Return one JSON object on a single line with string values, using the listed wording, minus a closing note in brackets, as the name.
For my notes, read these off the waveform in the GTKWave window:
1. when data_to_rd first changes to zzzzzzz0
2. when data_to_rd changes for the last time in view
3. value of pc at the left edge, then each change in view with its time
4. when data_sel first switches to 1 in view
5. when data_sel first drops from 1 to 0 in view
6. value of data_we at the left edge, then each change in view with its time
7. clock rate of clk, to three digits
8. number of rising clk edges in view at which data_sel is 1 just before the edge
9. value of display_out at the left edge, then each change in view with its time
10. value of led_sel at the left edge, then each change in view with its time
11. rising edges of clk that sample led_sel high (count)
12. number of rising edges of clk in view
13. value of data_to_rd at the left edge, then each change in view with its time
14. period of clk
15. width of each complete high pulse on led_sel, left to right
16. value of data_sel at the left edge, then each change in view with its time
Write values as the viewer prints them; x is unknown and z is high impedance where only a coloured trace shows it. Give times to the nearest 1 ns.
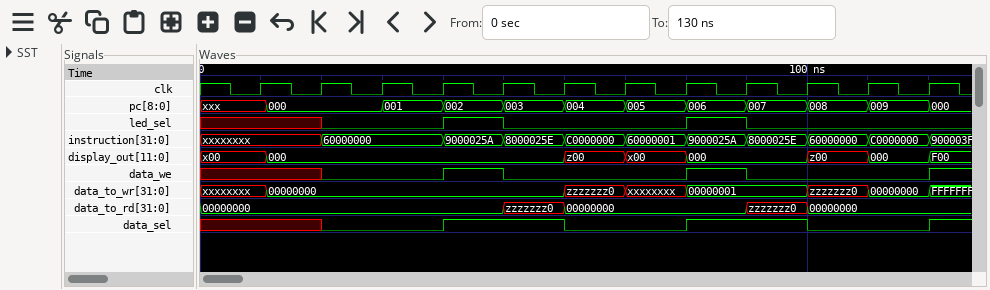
{"when data_to_rd first changes to zzzzzzz0": "50 ns", "when data_to_rd changes for the last time in view": "100 ns", "value of pc at the left edge, then each change in view with its time": "xxx, 000 at 11 ns, 001 at 30 ns, 002 at 40 ns, 003 at 50 ns, 004 at 60 ns, 005 at 70 ns, 006 at 80 ns, 007 at 90 ns, 008 at 100 ns, 009 at 110 ns, 000 at 120 ns", "when data_sel first switches to 1 in view": "40 ns", "when data_sel first drops from 1 to 0 in view": "60 ns", "value of data_we at the left edge, then each change in view with its time": "x, 0 at 20 ns, 1 at 40 ns, 0 at 50 ns, 1 at 80 ns, 0 at 90 ns, 1 at 120 ns", "clock rate of clk, to three digits": "100 MHz", "number of rising clk edges in view at which data_sel is 1 just before the edge": "4", "value of display_out at the left edge, then each change in view with its time": "x00, 000 at 11 ns, z00 at 60 ns, x00 at 70 ns, 000 at 80 ns, z00 at 100 ns, 000 at 110 ns, F00 at 120 ns", "value of led_sel at the left edge, then each change in view with its time": "x, 0 at 20 ns, 1 at 40 ns, 0 at 50 ns, 1 at 80 ns, 0 at 90 ns", "rising edges of clk that sample led_sel high": "2", "number of rising edges of clk in view": "12", "value of data_to_rd at the left edge, then each change in view with its time": "00000000, zzzzzzz0 at 50 ns, 00000000 at 60 ns, zzzzzzz0 at 90 ns, 00000000 at 100 ns", "period of clk": "10 ns", "width of each complete high pulse on led_sel, left to right": "10 ns, 10 ns", "value of data_sel at the left edge, then each change in view with its time": "x, 0 at 20 ns, 1 at 40 ns, 0 at 60 ns, 1 at 80 ns, 0 at 100 ns, 1 at 120 ns"}
